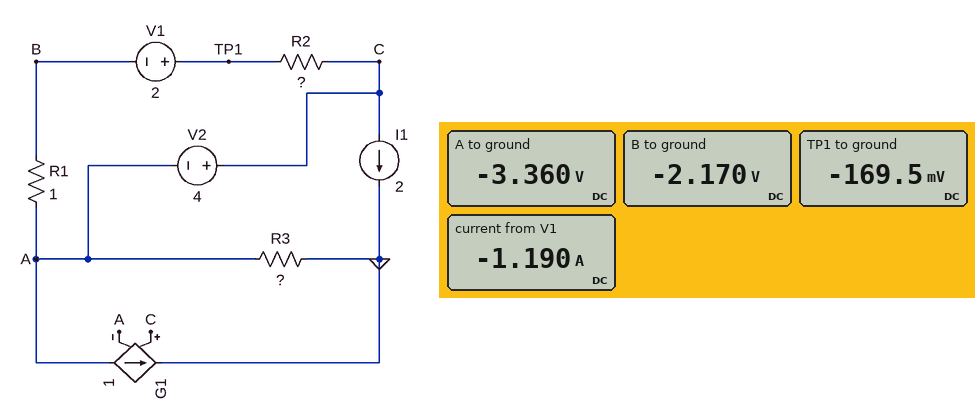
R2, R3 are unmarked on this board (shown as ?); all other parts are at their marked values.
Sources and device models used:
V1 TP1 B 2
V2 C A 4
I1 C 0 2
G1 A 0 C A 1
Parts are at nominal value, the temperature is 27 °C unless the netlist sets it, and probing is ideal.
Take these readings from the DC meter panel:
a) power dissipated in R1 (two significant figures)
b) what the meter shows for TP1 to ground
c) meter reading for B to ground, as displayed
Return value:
1.4 W
-169.5 mV
-2.170 V
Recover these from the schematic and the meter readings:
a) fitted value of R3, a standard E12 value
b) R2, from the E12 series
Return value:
0.56 Ω
0.68 Ω
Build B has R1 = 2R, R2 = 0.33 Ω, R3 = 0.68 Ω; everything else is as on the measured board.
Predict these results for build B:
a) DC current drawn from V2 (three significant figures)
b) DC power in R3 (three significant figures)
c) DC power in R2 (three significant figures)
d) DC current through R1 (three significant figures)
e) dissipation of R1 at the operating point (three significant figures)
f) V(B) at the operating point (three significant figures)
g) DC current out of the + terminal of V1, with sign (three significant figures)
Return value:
2.86 A
24.5 W
243 mW
858 mA
1.47 W
-2.36 V
-858 mA
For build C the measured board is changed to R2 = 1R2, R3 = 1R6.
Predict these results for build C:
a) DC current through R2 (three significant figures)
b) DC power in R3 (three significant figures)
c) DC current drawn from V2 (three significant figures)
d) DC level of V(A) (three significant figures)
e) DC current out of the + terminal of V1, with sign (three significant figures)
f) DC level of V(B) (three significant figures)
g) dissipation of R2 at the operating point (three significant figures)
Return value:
909 mA
57.6 W
2.91 A
-9.60 V
-909 mA
-8.69 V
992 mW
